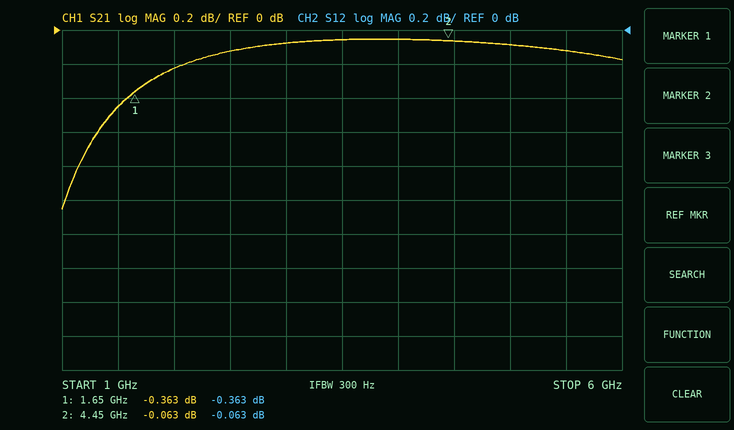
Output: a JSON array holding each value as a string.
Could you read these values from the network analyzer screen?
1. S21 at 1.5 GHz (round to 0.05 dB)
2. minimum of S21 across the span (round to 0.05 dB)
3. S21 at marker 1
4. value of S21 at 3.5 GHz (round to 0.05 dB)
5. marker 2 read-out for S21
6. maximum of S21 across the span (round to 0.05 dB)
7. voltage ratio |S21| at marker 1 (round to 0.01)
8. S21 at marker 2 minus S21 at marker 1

["-0.45 dB", "-1.05 dB", "-0.363 dB", "-0.05 dB", "-0.063 dB", "-0.05 dB", "0.96", "0.300 dB"]
